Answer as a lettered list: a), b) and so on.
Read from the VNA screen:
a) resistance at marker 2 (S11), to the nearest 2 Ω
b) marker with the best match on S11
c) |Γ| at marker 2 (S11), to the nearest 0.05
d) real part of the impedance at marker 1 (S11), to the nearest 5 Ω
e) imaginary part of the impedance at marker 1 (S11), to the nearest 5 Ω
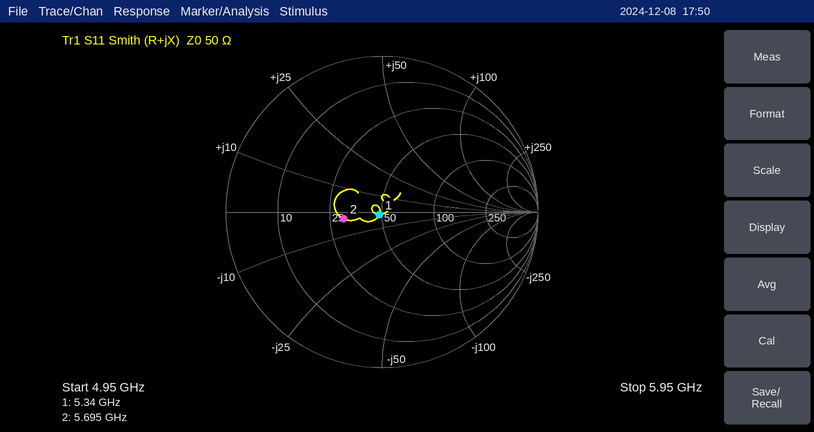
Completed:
a) 30 Ω
b) marker 1
c) 0.25
d) 50 Ω
e) 0 Ω
